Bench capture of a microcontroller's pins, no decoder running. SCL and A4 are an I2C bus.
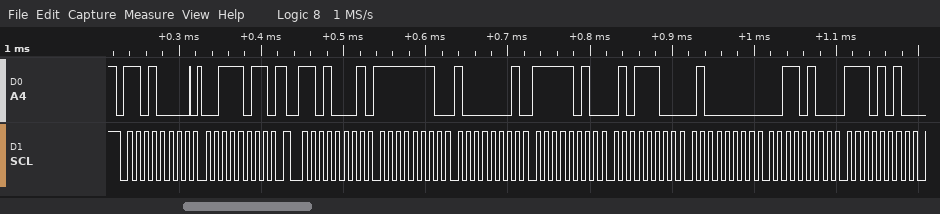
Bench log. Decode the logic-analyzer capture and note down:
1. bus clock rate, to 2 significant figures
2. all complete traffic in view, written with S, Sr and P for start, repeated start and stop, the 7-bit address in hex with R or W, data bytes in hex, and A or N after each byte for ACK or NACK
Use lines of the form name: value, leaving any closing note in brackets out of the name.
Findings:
bus clock rate, to 2 significant figures: 100 kHz
all complete traffic in view, written with S, Sr and P for start, repeated start and stop, the 7-bit address in hex with R or W, data bytes in hex, and A or N after each byte for ACK or NACK: S 68W A 3B A Sr 68R A FE A 81 A FA A 5C A 40 A 34 A EA A
